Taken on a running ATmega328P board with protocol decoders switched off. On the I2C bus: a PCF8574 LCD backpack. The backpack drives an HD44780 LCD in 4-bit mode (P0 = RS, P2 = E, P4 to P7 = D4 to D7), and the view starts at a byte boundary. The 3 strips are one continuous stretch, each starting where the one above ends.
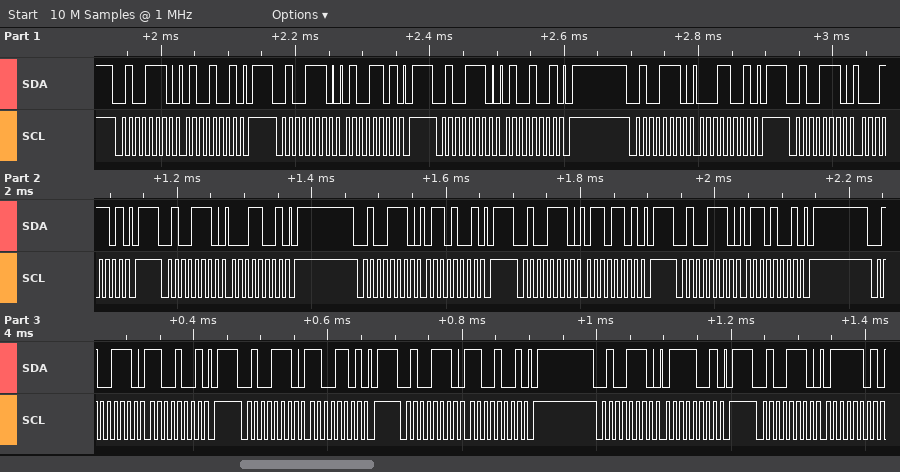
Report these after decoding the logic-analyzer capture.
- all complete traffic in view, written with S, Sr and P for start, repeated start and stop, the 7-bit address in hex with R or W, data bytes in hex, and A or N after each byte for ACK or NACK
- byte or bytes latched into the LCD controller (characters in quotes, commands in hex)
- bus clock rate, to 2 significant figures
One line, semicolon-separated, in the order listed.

S 27W A 49 A P S 27W A 4D A P S 27W A 49 A P S 27W A 19 A P S 27W A 1D A P S 27W A 19 A P S 27W A 69 A P S 27W A 6D A P S 27W A 69 A P S 27W A C9 A P S 27W A CD A P S 27W A C9 A P S 27W A 79 A P S 27W A 7D A; 'A' 'l'; 100 kHz
